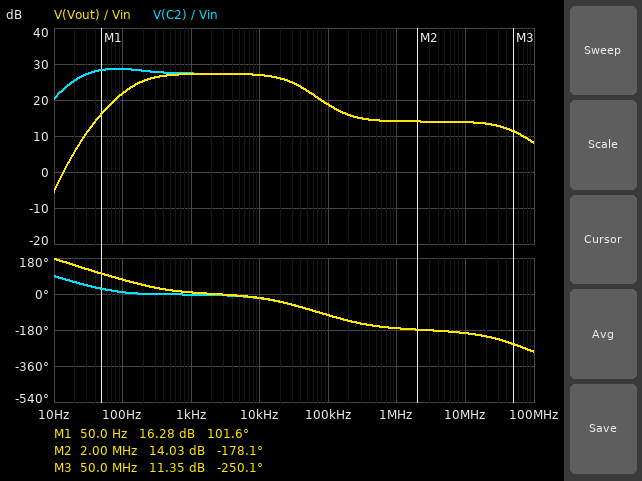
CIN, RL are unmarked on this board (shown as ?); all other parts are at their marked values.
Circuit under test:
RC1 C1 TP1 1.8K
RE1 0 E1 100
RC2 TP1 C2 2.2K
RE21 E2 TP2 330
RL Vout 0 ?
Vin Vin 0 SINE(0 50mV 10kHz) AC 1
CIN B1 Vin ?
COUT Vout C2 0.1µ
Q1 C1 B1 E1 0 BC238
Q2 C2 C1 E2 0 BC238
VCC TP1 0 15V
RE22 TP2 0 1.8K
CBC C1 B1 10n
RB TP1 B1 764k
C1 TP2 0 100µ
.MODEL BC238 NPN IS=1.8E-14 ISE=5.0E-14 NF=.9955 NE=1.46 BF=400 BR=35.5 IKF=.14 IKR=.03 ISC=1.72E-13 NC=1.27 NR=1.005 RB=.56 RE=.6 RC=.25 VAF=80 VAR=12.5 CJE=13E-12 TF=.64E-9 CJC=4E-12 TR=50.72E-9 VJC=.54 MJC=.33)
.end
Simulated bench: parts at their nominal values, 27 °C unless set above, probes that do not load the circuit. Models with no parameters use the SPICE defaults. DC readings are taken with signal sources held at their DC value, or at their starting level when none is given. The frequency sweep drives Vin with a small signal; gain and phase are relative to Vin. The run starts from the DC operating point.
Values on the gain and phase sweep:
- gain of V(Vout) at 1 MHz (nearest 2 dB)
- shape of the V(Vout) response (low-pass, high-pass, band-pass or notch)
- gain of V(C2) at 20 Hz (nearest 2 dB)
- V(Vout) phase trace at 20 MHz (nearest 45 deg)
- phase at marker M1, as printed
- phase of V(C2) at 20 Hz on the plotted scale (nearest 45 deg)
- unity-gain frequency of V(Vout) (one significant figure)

14 dB
band-pass
26 dB
-225 deg
101.6 deg
45 deg
10 Hz
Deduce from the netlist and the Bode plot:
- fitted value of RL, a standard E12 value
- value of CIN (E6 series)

8.2 kΩ
68 nF
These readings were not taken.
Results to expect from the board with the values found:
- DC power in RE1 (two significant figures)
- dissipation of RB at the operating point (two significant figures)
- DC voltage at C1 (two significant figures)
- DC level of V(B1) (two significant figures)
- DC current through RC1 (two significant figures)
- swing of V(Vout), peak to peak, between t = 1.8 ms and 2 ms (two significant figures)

3.1 mW
250 µW
5.0 V
1.2 V
5.5 mA
2.2 V
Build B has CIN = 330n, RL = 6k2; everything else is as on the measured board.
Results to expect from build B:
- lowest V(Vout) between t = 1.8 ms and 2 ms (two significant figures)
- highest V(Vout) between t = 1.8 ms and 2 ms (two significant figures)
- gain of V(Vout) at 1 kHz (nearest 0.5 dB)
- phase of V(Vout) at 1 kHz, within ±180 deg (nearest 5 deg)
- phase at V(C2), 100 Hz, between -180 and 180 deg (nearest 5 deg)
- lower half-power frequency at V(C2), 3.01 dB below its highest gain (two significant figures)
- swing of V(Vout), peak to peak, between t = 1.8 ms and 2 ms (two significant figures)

-2.1 V
2.0 V
34.0 dB
5 deg
0 deg
12 Hz
4.1 V
